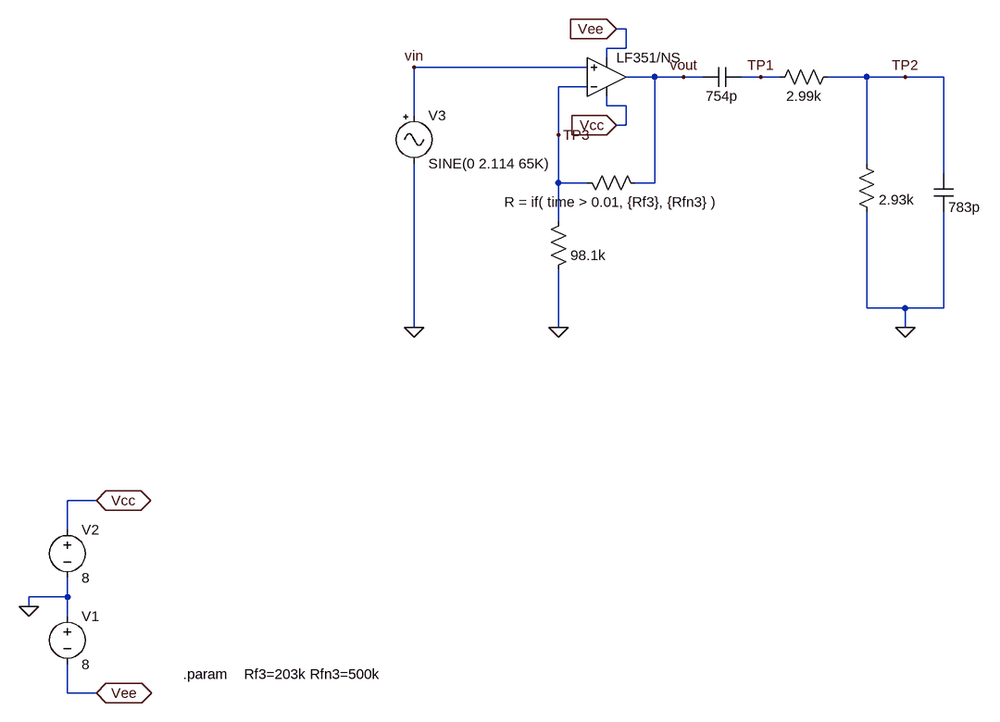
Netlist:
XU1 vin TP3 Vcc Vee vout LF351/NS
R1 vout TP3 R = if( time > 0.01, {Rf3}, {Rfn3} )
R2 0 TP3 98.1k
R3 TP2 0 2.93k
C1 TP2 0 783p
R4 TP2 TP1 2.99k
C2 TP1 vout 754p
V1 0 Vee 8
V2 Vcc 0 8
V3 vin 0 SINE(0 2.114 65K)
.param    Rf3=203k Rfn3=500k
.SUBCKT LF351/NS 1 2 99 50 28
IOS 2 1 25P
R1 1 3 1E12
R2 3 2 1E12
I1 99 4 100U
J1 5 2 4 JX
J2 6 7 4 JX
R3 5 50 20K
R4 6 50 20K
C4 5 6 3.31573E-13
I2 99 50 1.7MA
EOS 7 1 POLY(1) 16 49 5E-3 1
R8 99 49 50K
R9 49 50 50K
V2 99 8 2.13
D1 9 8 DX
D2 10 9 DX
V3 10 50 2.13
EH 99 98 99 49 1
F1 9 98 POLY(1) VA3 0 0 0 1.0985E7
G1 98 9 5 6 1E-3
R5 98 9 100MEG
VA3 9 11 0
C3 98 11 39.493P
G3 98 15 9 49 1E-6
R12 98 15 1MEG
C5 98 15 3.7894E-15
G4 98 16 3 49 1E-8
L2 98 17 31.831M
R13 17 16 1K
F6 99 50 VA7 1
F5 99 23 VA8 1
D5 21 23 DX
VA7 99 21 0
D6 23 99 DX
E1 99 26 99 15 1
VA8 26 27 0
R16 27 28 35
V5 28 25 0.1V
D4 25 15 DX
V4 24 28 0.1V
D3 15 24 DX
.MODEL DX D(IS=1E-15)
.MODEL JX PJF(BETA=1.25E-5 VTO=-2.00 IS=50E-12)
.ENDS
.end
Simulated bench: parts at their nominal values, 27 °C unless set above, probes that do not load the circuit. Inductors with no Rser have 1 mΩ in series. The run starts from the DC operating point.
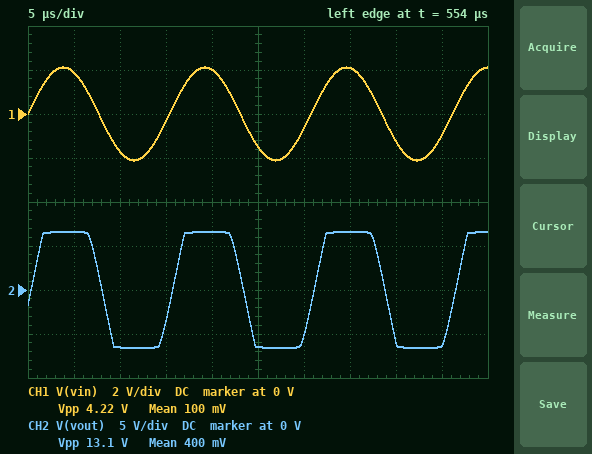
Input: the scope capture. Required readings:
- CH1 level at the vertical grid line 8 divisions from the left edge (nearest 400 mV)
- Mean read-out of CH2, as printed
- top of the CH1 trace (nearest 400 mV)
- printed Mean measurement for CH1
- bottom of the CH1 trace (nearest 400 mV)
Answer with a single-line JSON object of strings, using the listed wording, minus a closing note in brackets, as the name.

{"CH1 level at the vertical grid line 8 divisions from the left edge": "-1.2 V", "Mean read-out of CH2, as printed": "400 mV", "top of the CH1 trace": "2.0 V", "printed Mean measurement for CH1": "100 mV", "bottom of the CH1 trace": "-2.0 V"}
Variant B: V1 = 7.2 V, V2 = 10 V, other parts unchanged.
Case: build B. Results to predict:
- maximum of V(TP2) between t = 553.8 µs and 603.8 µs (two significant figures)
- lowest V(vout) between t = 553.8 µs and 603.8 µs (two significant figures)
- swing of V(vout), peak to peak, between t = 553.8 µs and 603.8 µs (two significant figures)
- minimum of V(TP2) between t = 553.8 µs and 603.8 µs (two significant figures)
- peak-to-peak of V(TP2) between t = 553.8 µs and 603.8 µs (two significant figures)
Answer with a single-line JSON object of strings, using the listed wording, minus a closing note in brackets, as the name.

{"maximum of V(TP2) between t = 553.8 µs and 603.8 µs": "2.8 V", "lowest V(vout) between t = 553.8 µs and 603.8 µs": "-5.8 V", "swing of V(vout), peak to peak, between t = 553.8 µs and 603.8 µs": "14 V", "minimum of V(TP2) between t = 553.8 µs and 603.8 µs": "-2.6 V", "peak-to-peak of V(TP2) between t = 553.8 µs and 603.8 µs": "5.4 V"}
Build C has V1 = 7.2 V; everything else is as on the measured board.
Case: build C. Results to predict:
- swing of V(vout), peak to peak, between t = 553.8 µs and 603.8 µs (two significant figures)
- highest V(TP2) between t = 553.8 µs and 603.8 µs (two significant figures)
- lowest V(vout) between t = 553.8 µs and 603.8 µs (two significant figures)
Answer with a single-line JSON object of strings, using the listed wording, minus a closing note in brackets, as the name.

{"swing of V(vout), peak to peak, between t = 553.8 µs and 603.8 µs": "12 V", "highest V(TP2) between t = 553.8 µs and 603.8 µs": "2.4 V", "lowest V(vout) between t = 553.8 µs and 603.8 µs": "-5.8 V"}
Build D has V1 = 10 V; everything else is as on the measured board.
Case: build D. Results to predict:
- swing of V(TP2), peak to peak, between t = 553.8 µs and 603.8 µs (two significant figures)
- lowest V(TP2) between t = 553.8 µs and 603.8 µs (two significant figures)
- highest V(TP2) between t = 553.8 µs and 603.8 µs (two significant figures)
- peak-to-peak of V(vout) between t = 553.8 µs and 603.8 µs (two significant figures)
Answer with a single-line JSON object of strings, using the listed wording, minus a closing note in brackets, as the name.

{"swing of V(TP2), peak to peak, between t = 553.8 µs and 603.8 µs": "5.7 V", "lowest V(TP2) between t = 553.8 µs and 603.8 µs": "-2.9 V", "highest V(TP2) between t = 553.8 µs and 603.8 µs": "2.8 V", "peak-to-peak of V(vout) between t = 553.8 µs and 603.8 µs": "15 V"}
